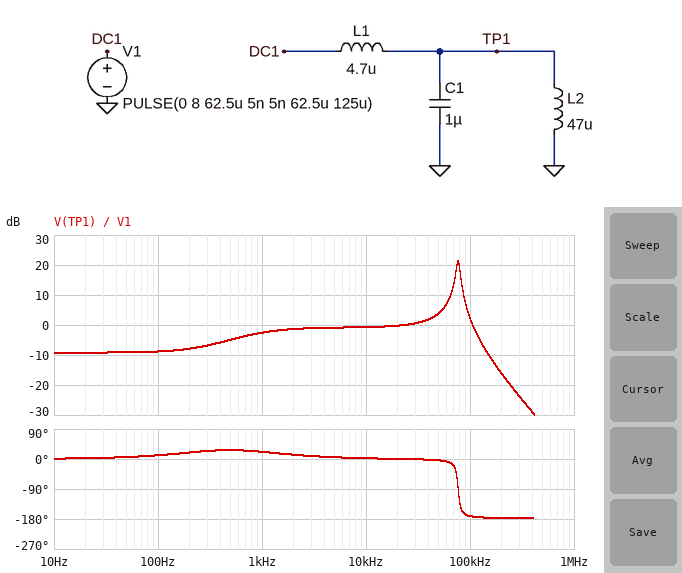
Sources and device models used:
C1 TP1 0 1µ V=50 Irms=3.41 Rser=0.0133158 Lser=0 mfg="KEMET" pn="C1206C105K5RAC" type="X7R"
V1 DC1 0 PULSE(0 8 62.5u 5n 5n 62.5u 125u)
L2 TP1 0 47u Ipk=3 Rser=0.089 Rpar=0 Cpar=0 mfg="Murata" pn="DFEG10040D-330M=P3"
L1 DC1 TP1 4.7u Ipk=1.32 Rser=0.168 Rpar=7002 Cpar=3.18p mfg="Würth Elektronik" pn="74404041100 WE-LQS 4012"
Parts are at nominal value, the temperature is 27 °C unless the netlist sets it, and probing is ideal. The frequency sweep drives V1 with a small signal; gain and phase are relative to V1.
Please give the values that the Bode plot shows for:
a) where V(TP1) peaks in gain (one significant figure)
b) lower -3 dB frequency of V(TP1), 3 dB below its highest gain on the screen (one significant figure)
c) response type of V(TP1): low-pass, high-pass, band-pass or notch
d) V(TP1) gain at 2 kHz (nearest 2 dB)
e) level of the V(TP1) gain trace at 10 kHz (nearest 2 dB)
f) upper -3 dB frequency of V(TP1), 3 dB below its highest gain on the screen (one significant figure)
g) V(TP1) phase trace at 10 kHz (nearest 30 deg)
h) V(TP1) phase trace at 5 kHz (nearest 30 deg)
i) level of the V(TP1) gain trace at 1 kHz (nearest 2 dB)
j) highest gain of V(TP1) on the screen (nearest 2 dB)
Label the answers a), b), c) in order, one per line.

a) 80 kHz
b) 70 kHz
c) band-pass
d) -2 dB
e) 0 dB
f) 80 kHz
g) 0 deg
h) 0 deg
i) -2 dB
j) 22 dB
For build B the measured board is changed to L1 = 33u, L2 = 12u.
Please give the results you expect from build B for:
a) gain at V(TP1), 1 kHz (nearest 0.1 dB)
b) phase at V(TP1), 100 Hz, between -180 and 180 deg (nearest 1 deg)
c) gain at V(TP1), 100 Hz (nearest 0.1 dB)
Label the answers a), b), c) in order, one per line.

a) -10.3 dB
b) -1 deg
c) -9.2 dB
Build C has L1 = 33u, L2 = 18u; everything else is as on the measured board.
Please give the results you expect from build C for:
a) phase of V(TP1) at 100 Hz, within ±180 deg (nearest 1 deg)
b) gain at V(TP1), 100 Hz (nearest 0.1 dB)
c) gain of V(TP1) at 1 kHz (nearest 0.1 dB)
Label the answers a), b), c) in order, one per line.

a) 0 deg
b) -9.2 dB
c) -9.1 dB
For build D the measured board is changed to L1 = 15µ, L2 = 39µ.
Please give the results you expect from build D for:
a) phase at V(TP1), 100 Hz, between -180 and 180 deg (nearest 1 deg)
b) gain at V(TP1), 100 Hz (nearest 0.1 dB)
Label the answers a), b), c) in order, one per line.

a) 8 deg
b) -9.0 dB
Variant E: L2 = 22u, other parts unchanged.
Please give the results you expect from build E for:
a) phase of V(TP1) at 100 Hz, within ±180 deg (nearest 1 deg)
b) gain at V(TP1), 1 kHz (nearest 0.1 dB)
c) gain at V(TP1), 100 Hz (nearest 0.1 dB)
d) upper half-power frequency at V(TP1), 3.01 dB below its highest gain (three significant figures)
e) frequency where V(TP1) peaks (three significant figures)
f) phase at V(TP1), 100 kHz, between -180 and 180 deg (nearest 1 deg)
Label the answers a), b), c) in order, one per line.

a) 5 deg
b) -5.4 dB
c) -9.1 dB
d) 83.4 kHz
e) 80.8 kHz
f) -170 deg
